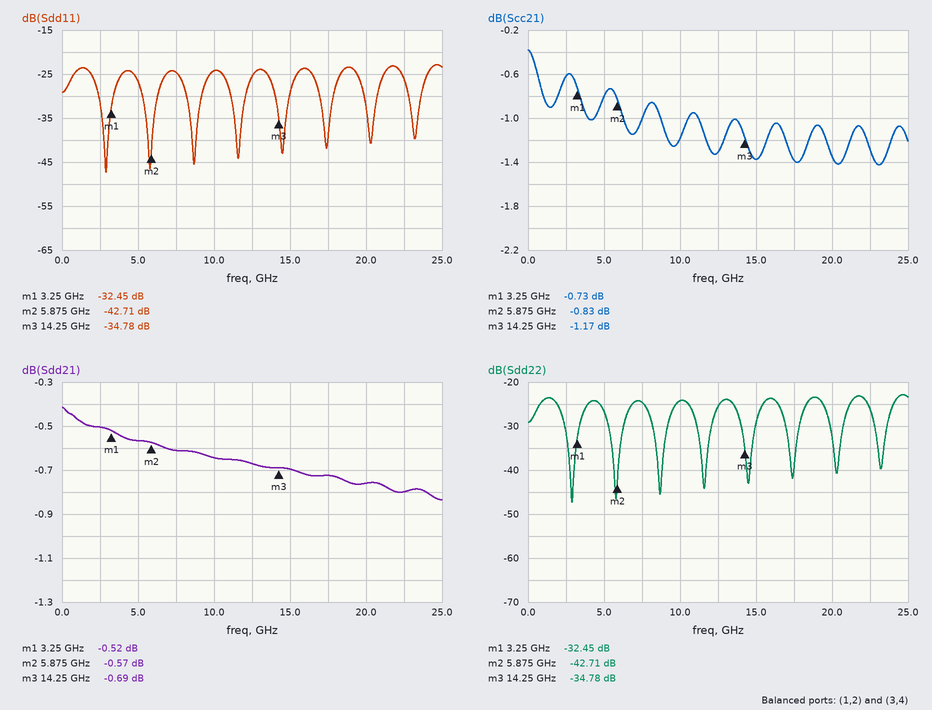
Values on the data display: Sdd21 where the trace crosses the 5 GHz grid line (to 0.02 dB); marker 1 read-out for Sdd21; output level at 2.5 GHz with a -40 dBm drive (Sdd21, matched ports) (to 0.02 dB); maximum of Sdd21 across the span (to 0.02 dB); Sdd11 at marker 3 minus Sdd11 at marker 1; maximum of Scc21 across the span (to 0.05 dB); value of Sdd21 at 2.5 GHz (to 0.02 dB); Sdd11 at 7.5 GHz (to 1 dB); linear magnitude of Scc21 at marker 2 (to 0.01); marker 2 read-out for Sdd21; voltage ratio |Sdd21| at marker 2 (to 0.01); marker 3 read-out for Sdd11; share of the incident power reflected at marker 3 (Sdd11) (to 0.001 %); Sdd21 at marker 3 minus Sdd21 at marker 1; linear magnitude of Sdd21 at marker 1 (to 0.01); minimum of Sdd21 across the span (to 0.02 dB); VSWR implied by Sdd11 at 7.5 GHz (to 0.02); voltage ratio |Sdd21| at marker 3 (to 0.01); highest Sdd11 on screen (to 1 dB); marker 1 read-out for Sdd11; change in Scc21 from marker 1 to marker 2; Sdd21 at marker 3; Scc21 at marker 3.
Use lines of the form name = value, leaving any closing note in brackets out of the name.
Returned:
Sdd21 where the trace crosses the 5 GHz grid line = -0.56 dB
marker 1 read-out for Sdd21 = -0.52 dB
output level at 2.5 GHz with a -40 dBm drive (Sdd21, matched ports) = -40.50 dBm
maximum of Sdd21 across the span = -0.42 dB
Sdd11 at marker 3 minus Sdd11 at marker 1 = -2.33 dB
maximum of Scc21 across the span = -0.40 dB
value of Sdd21 at 2.5 GHz = -0.50 dB
Sdd11 at 7.5 GHz = -25 dB
linear magnitude of Scc21 at marker 2 = 0.91
marker 2 read-out for Sdd21 = -0.57 dB
voltage ratio |Sdd21| at marker 2 = 0.94
marker 3 read-out for Sdd11 = -34.78 dB
share of the incident power reflected at marker 3 (Sdd11) = 0.033 %
Sdd21 at marker 3 minus Sdd21 at marker 1 = -0.17 dB
linear magnitude of Sdd21 at marker 1 = 0.94
minimum of Sdd21 across the span = -0.84 dB
VSWR implied by Sdd11 at 7.5 GHz = 1.12
voltage ratio |Sdd21| at marker 3 = 0.92
highest Sdd11 on screen = -23 dB
marker 1 read-out for Sdd11 = -32.45 dB
change in Scc21 from marker 1 to marker 2 = -0.10 dB
Sdd21 at marker 3 = -0.69 dB
Scc21 at marker 3 = -1.17 dB
